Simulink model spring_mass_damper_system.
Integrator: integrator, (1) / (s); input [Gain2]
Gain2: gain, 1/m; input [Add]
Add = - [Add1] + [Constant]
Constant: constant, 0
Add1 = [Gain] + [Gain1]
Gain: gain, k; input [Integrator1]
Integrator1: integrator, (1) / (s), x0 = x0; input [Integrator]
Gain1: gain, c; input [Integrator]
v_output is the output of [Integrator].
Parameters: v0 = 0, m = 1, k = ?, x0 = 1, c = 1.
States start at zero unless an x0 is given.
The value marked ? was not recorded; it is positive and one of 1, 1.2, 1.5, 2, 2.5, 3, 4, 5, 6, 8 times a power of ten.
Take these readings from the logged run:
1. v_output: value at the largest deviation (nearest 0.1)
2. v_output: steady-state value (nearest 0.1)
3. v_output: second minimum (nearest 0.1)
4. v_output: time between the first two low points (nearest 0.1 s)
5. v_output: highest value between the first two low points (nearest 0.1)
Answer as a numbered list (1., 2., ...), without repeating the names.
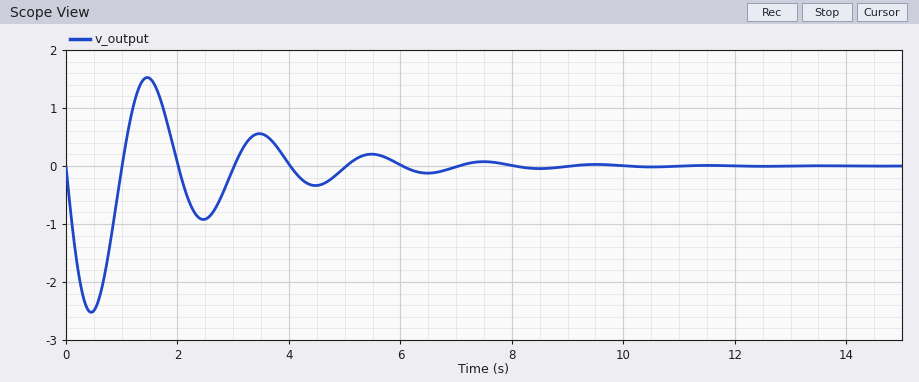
1. -2.5
2. 0.0
3. -0.9
4. 2.0 s
5. 1.5
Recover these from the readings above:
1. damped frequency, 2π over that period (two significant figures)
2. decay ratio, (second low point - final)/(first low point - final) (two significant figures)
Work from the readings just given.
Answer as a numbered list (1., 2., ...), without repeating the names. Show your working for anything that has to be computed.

1. 2π / 2 = 3.1 rad/s
2. (-0.9 - 0) / (-2.5 - 0) = 0.36
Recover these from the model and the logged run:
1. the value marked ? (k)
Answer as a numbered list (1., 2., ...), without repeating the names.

1. 10
